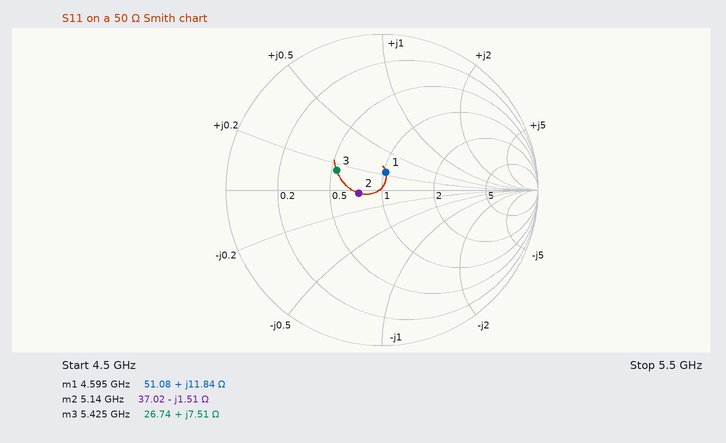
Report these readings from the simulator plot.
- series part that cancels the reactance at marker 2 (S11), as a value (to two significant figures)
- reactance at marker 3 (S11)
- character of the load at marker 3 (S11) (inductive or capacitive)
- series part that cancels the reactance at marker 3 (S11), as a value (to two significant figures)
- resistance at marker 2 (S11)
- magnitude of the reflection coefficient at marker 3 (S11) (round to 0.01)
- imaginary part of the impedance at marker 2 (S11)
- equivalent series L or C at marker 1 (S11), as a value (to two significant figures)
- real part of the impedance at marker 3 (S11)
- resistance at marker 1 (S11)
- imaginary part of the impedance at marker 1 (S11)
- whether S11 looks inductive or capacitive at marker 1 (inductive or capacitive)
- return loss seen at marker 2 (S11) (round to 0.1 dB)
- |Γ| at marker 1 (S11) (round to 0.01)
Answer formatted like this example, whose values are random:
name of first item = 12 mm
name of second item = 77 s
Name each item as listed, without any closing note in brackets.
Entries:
series part that cancels the reactance at marker 2 (S11), as a value = 47 pH
reactance at marker 3 = +7.51 Ω
character of the load at marker 3 (S11) = inductive
series part that cancels the reactance at marker 3 (S11), as a value = 3.9 pF
resistance at marker 2 = 37.02 Ω
magnitude of the reflection coefficient at marker 3 (S11) = 0.32
imaginary part of the impedance at marker 2 = -1.51 Ω
equivalent series L or C at marker 1 (S11), as a value = 410 pH
real part of the impedance at marker 3 = 26.74 Ω
resistance at marker 1 = 51.08 Ω
imaginary part of the impedance at marker 1 = +11.84 Ω
whether S11 looks inductive or capacitive at marker 1 = inductive
return loss seen at marker 2 (S11) = 16.5 dB
|Γ| at marker 1 (S11) = 0.12
